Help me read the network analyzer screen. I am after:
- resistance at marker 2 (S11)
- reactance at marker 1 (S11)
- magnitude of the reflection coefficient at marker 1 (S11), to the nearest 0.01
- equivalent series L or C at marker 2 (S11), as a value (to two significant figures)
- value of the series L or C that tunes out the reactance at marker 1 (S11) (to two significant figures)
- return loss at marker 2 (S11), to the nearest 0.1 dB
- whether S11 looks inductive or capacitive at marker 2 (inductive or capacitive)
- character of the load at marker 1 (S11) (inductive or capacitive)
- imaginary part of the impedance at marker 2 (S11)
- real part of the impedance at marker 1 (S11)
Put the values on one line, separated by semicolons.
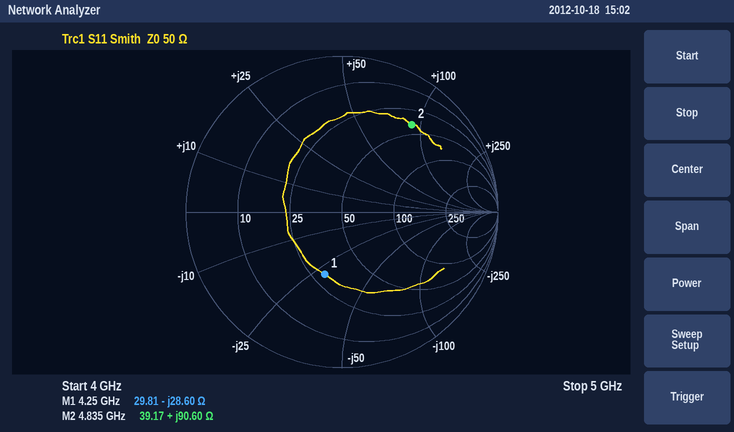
39.17 Ω; -28.60 Ω; 0.41; 3.0 nH; 1.1 nH; 2.9 dB; inductive; capacitive; +90.60 Ω; 29.81 Ω
